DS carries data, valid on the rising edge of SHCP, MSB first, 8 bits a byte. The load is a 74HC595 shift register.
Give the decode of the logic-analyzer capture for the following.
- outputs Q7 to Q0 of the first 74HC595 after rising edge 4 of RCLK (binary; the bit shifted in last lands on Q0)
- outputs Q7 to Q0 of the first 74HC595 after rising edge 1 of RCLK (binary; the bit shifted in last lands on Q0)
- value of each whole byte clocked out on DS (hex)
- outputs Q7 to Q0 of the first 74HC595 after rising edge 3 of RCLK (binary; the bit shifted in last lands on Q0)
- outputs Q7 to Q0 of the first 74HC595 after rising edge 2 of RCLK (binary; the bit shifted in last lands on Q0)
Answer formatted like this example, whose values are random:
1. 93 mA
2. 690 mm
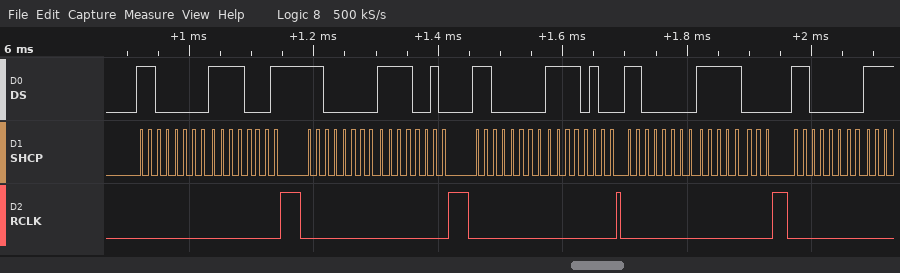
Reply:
1. 11111000
2. 11110001
3. C0 F1 C0 F2 C0 F4 C0 F8 C0
4. 11110100
5. 11110010
